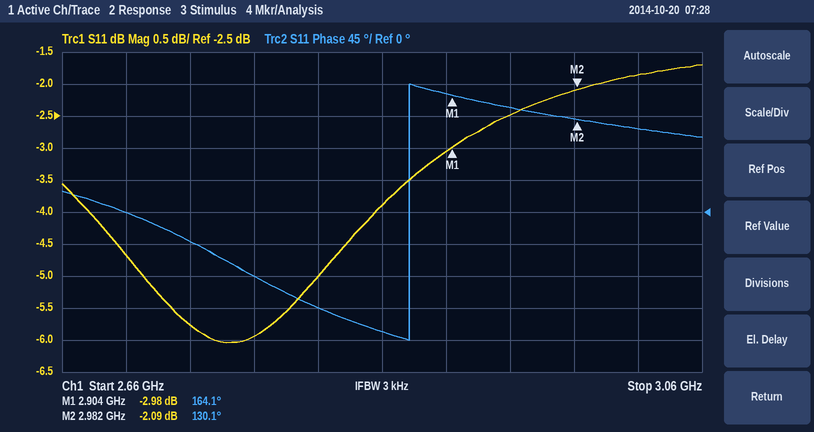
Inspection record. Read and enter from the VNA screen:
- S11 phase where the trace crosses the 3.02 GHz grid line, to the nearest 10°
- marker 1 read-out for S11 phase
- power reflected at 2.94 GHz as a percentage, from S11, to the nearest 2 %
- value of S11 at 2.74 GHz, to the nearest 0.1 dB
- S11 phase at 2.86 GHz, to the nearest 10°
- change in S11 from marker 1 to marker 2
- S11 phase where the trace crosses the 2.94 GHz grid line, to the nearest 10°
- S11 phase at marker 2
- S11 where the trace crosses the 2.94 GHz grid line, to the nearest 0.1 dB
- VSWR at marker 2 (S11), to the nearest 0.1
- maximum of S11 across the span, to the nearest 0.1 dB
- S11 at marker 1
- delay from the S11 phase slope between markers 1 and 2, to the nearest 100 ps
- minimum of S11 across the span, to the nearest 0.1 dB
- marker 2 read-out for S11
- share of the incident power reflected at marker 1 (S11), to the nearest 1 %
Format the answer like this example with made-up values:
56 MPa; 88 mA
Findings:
120°; 164.1°; 56 %; -5.8 dB; -170°; 0.89 dB; 150°; 130.1°; -2.5 dB; 8.4; -1.7 dB; -2.98 dB; 1.2 ns; -6.0 dB; -2.09 dB; 50 %
